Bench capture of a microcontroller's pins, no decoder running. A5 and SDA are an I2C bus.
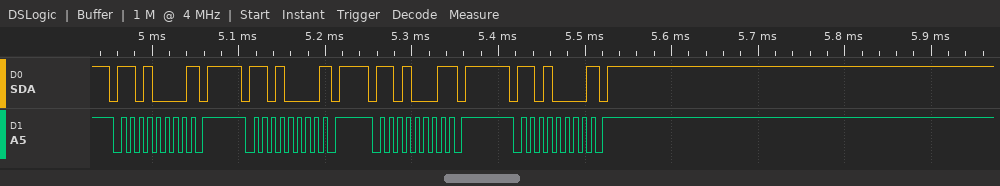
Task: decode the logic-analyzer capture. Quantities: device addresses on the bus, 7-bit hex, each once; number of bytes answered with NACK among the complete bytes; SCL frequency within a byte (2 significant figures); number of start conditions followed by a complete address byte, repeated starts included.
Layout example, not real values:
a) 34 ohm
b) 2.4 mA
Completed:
a) 0x68
b) 4
c) 100 kHz
d) 4
